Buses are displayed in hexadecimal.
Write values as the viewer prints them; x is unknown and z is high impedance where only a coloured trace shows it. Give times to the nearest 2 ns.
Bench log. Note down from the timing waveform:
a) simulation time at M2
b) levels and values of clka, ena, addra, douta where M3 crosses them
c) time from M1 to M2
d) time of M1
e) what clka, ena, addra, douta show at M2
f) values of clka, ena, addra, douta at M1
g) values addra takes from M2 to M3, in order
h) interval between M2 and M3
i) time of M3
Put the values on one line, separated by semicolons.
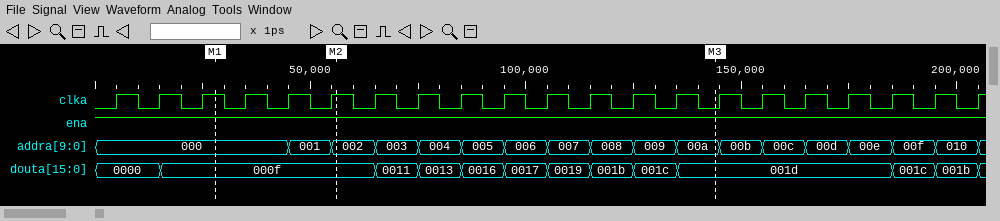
56 ns; clka=0, ena=1, addra=00a, douta=001d; 28 ns; 28 ns; clka=1, ena=1, addra=002, douta=000f; clka=1, ena=1, addra=000, douta=000f; 002, 003, 004, 005, 006, 007, 008, 009, 00a; 88 ns; 144 ns
